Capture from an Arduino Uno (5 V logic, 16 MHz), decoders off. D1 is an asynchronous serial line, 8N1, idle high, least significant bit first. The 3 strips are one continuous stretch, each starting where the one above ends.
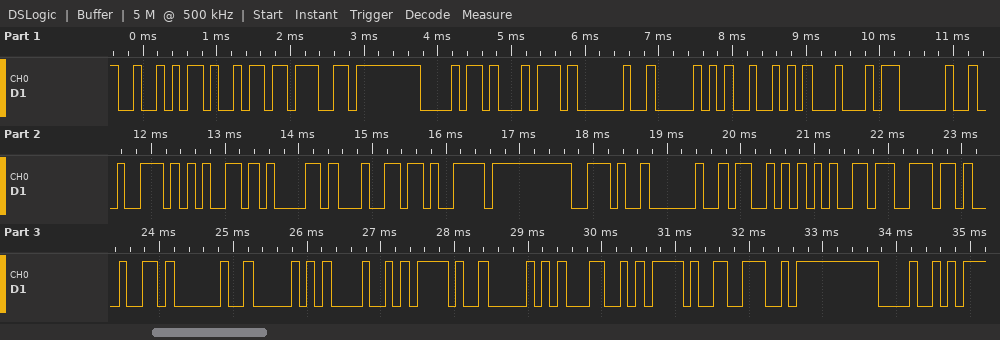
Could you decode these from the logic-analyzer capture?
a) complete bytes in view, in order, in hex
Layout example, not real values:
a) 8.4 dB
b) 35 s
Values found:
a) 52 69 67 68 74 20 50 52 44 20 72 65 61 64 79 2E 20 53 65 6E 64 20 50 48 2F 50 4C 2F 4E 48
